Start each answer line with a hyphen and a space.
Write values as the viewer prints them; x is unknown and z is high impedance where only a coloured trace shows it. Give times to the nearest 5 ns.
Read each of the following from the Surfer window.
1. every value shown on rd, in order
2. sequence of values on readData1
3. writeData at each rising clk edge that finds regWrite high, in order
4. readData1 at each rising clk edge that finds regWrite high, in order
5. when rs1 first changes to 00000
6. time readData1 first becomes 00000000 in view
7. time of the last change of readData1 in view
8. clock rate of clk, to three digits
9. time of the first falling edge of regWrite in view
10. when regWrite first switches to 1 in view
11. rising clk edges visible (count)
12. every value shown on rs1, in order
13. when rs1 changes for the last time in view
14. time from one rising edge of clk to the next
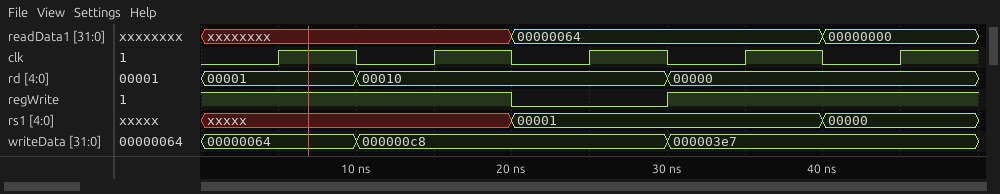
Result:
- 00001, 00010, 00000
- xxxxxxxx, 00000064, 00000000
- 00000064, 000000c8, 000003e7, 000003e7
- xxxxxxxx, xxxxxxxx, 00000064, 00000000
- 40 ns
- 40 ns
- 40 ns
- 100 MHz
- 20 ns
- 30 ns
- 5
- xxxxx, 00001, 00000
- 40 ns
- 10 ns
